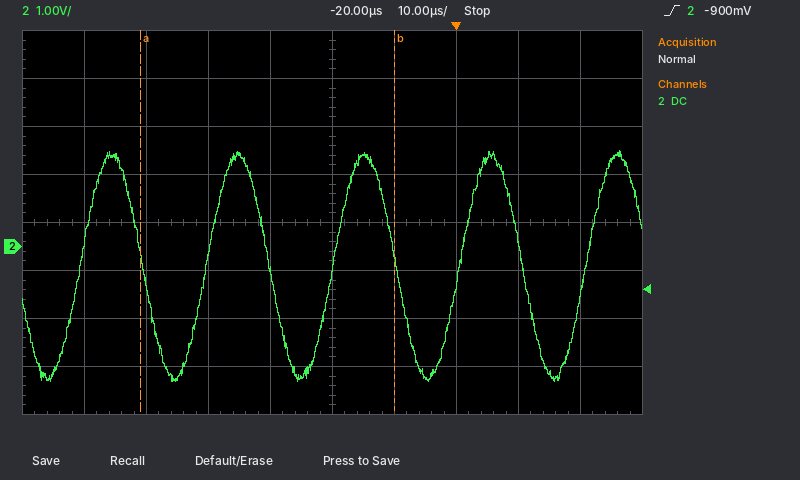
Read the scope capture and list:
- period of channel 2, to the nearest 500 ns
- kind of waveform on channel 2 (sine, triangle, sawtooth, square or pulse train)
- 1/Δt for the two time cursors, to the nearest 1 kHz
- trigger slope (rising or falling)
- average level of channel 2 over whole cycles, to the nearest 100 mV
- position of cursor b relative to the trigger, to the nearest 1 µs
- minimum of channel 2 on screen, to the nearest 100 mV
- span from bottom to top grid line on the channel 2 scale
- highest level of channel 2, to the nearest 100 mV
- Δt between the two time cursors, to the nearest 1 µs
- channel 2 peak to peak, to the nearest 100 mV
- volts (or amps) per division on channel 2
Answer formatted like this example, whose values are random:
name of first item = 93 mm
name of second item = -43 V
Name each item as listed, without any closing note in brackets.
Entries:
period of channel 2, to the nearest 500 ns = 20.5 µs
kind of waveform on channel 2 = sine
1/Δt for the two time cursors, to the nearest 1 kHz = 24 kHz
trigger slope = rising
average level of channel 2 over whole cycles, to the nearest 100 mV = -400 mV
position of cursor b relative to the trigger, to the nearest 1 µs = -10 µs
minimum of channel 2 on screen, to the nearest 100 mV = -2.8 V
span from bottom to top grid line on the channel 2 scale = 8 V
highest level of channel 2, to the nearest 100 mV = 2.0 V
Δt between the two time cursors, to the nearest 1 µs = 41 µs
channel 2 peak to peak, to the nearest 100 mV = 4.8 V
volts (or amps) per division on channel 2 = 1 V
